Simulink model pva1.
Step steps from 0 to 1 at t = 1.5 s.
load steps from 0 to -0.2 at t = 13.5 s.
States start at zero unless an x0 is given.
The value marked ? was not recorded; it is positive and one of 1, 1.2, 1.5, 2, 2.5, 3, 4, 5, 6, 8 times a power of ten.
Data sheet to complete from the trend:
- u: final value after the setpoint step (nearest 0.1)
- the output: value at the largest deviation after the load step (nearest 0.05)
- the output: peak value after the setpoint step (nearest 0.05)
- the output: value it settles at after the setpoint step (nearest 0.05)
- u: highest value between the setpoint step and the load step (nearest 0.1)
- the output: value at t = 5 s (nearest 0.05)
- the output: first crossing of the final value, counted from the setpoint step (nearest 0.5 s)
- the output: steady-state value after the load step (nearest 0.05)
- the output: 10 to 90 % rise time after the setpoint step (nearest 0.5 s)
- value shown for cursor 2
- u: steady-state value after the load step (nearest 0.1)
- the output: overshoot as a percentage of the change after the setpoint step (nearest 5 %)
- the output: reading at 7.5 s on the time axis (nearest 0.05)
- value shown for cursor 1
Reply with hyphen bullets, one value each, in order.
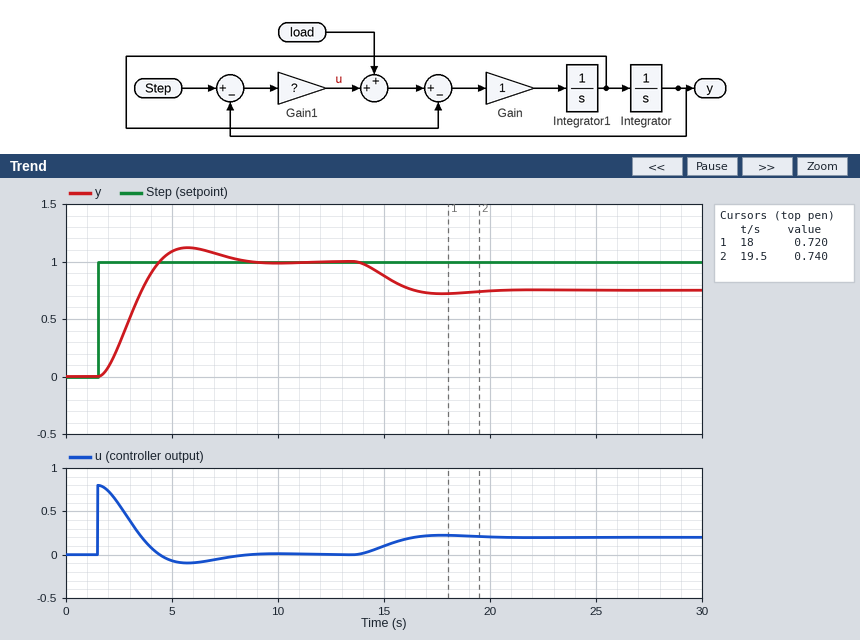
- 0.0
- 0.70
- 1.10
- 1.00
- 0.8
- 1.10
- 3.0 s
- 0.75
- 2.0 s
- 0.740
- 0.2
- 10 %
- 1.05
- 0.720
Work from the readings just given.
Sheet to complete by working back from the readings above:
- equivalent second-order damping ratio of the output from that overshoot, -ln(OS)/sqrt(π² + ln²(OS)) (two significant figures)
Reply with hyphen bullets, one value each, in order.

- 0.59
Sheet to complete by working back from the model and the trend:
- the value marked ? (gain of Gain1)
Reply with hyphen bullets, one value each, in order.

- 0.8
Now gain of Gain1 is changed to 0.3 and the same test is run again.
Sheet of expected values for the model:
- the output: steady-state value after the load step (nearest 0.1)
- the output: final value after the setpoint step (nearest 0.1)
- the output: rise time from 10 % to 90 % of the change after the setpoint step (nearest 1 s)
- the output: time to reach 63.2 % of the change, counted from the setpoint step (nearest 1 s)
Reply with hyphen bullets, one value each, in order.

- 0.3
- 1.0
- 5 s
- 4 s
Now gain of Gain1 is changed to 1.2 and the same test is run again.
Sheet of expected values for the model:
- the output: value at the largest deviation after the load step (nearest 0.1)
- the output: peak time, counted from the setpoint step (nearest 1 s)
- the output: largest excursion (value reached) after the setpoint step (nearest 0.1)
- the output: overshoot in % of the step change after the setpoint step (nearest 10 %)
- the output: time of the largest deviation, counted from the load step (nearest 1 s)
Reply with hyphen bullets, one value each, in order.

- 0.8
- 3 s
- 1.2
- 20 %
- 3 s
